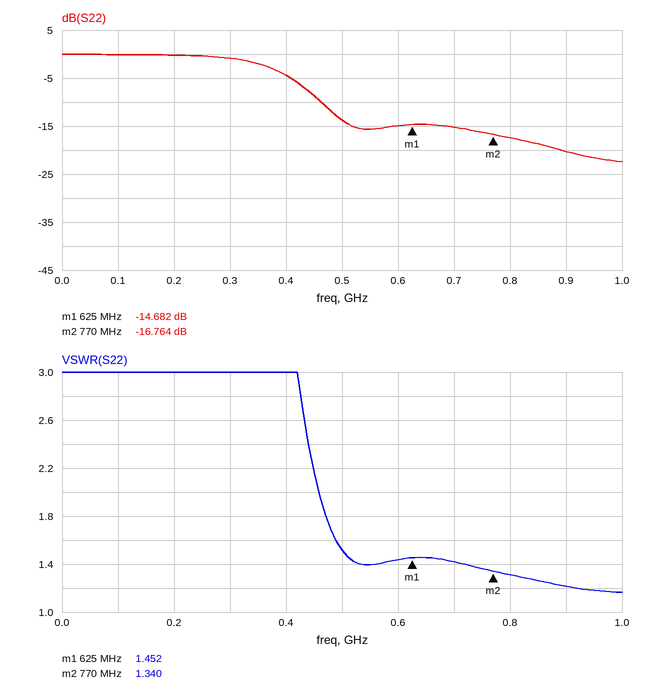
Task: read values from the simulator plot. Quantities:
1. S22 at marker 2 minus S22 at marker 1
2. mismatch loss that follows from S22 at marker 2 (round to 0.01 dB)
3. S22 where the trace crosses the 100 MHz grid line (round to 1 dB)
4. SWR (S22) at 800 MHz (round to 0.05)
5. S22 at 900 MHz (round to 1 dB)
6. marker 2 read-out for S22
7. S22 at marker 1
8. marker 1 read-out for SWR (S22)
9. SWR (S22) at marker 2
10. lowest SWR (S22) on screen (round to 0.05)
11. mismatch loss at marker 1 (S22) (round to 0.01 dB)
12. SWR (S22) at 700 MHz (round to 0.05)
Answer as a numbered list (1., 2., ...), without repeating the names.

1. -2.082 dB
2. 0.09 dB
3. 0 dB
4. 1.30
5. -20 dB
6. -16.764 dB
7. -14.682 dB
8. 1.452
9. 1.340
10. 1.15
11. 0.15 dB
12. 1.40
